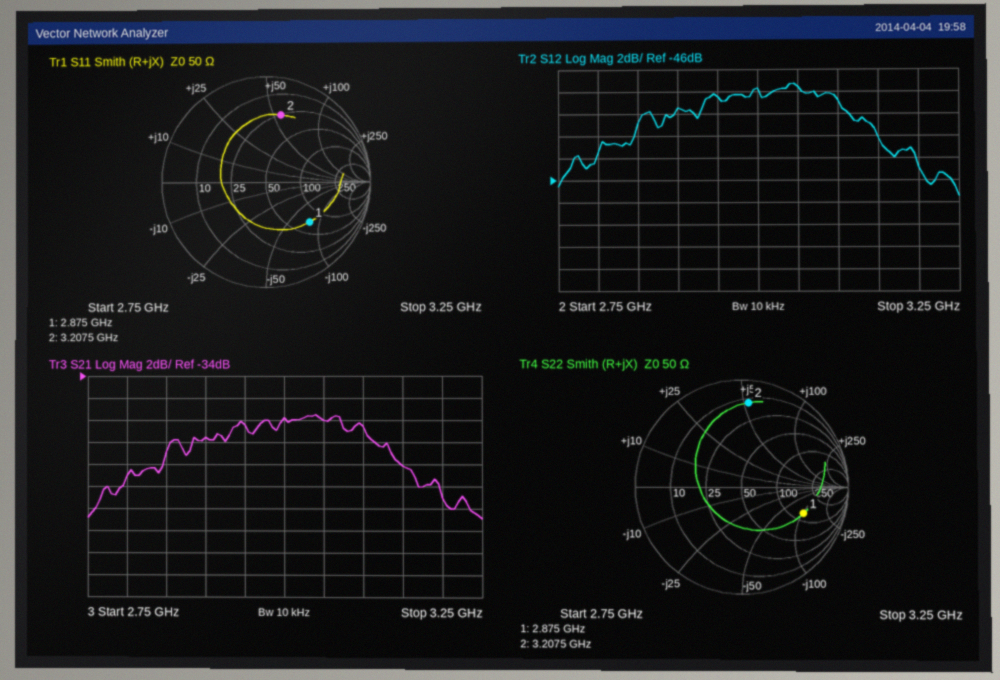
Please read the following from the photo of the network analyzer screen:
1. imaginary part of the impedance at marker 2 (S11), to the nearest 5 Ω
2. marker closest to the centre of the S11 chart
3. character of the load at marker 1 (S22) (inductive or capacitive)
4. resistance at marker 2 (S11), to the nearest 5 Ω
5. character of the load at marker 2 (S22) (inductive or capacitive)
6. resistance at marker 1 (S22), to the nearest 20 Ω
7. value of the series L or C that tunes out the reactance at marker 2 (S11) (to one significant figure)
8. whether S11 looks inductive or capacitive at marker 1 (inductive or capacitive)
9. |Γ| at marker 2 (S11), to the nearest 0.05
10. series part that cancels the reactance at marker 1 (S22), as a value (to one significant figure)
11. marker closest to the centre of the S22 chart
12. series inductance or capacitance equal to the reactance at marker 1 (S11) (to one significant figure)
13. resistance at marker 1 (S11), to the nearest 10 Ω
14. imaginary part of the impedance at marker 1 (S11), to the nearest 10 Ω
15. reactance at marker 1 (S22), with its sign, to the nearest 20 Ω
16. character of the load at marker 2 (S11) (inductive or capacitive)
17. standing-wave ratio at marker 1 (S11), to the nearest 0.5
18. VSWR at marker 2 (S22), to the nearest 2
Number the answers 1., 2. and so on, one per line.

1. +55 Ω
2. marker 1
3. capacitive
4. 25 Ω
5. inductive
6. 120 Ω
7. 900 fF
8. capacitive
9. 0.65
10. 6 nH
11. marker 1
12. 700 fF
13. 70 Ω
14. -80 Ω
15. -100 Ω
16. inductive
17. 3.5
18. 8
